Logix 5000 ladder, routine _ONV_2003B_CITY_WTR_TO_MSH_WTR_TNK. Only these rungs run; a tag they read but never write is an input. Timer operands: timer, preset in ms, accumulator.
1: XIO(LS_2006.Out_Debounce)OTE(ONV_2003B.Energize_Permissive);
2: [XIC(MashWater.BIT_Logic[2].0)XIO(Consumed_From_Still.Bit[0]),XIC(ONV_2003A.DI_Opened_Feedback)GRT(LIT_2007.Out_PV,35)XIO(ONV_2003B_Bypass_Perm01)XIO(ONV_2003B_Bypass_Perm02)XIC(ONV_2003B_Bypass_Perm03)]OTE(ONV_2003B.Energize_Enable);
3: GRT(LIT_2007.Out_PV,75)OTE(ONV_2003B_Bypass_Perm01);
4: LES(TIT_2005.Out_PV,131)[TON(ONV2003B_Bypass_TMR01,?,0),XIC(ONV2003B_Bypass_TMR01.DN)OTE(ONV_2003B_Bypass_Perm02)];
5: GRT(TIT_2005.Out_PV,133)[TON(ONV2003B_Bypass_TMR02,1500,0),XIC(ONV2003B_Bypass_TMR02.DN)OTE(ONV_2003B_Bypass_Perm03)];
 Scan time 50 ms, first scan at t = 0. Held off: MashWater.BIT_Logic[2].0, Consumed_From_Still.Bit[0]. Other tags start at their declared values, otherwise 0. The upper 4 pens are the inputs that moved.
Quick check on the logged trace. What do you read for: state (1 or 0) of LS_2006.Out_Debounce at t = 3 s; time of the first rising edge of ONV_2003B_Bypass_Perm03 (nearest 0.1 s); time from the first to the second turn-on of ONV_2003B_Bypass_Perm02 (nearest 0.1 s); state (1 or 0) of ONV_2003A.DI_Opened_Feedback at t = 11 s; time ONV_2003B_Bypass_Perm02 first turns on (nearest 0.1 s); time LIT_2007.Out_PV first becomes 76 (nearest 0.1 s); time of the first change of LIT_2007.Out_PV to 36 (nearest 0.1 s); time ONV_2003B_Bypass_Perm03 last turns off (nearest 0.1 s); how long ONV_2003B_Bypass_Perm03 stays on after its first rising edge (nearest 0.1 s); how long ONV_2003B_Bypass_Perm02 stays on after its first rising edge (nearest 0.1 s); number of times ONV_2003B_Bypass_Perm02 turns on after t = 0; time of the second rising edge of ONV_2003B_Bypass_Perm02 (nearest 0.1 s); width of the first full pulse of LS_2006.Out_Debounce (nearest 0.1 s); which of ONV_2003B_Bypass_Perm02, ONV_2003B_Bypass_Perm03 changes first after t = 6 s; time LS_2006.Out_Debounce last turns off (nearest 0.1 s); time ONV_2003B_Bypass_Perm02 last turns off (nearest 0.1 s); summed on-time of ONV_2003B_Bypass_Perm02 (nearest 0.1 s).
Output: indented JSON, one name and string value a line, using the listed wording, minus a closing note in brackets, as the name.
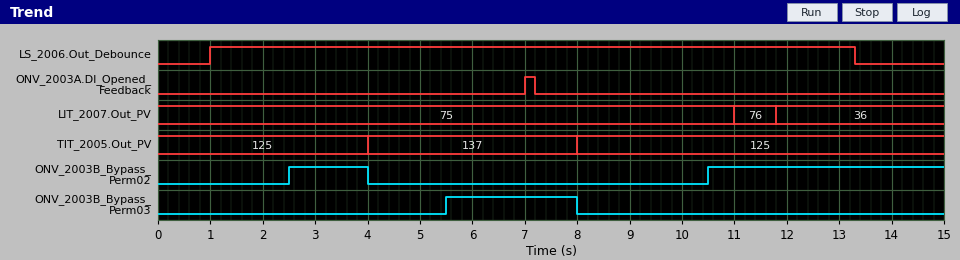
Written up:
{
  "state (1 or 0) of LS_2006.Out_Debounce at t = 3 s": "1",
  "time of the first rising edge of ONV_2003B_Bypass_Perm03": "5.5 s",
  "time from the first to the second turn-on of ONV_2003B_Bypass_Perm02": "8.0 s",
  "state (1 or 0) of ONV_2003A.DI_Opened_Feedback at t = 11 s": "0",
  "time ONV_2003B_Bypass_Perm02 first turns on": "2.5 s",
  "time LIT_2007.Out_PV first becomes 76": "11.0 s",
  "time of the first change of LIT_2007.Out_PV to 36": "11.8 s",
  "time ONV_2003B_Bypass_Perm03 last turns off": "8.0 s",
  "how long ONV_2003B_Bypass_Perm03 stays on after its first rising edge": "2.5 s",
  "how long ONV_2003B_Bypass_Perm02 stays on after its first rising edge": "1.5 s",
  "number of times ONV_2003B_Bypass_Perm02 turns on after t = 0": "2",
  "time of the second rising edge of ONV_2003B_Bypass_Perm02": "10.5 s",
  "width of the first full pulse of LS_2006.Out_Debounce": "12.3 s",
  "which of ONV_2003B_Bypass_Perm02, ONV_2003B_Bypass_Perm03 changes first after t = 6 s": "ONV_2003B_Bypass_Perm03",
  "time LS_2006.Out_Debounce last turns off": "13.3 s",
  "time ONV_2003B_Bypass_Perm02 last turns off": "4.0 s",
  "summed on-time of ONV_2003B_Bypass_Perm02": "6.0 s"
}
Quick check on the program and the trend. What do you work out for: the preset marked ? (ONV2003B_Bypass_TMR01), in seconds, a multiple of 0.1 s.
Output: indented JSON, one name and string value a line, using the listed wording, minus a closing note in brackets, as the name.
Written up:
{
  "the preset marked ? (ONV2003B_Bypass_TMR01), in seconds, a multiple of 0.1 s": "2.5 s"
}
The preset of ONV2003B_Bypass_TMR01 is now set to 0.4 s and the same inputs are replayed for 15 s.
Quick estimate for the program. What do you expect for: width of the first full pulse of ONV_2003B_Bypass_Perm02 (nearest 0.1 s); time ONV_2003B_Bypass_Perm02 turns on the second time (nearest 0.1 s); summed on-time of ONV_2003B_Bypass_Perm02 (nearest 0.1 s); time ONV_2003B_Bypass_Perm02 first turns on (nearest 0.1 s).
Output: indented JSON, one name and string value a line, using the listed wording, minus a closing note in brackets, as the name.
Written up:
{
  "width of the first full pulse of ONV_2003B_Bypass_Perm02": "3.6 s",
  "time ONV_2003B_Bypass_Perm02 turns on the second time": "8.4 s",
  "summed on-time of ONV_2003B_Bypass_Perm02": "10.2 s",
  "time ONV_2003B_Bypass_Perm02 first turns on": "0.4 s"
}
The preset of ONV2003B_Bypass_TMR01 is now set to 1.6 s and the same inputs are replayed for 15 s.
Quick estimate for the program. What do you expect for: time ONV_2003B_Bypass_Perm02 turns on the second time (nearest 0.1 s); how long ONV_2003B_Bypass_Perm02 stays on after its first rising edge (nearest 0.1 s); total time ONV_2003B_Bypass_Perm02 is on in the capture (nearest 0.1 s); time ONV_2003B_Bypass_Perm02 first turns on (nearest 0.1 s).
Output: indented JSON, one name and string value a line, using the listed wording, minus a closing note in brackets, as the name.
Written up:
{
  "time ONV_2003B_Bypass_Perm02 turns on the second time": "9.6 s",
  "how long ONV_2003B_Bypass_Perm02 stays on after its first rising edge": "2.4 s",
  "total time ONV_2003B_Bypass_Perm02 is on in the capture": "7.8 s",
  "time ONV_2003B_Bypass_Perm02 first turns on": "1.6 s"
}
